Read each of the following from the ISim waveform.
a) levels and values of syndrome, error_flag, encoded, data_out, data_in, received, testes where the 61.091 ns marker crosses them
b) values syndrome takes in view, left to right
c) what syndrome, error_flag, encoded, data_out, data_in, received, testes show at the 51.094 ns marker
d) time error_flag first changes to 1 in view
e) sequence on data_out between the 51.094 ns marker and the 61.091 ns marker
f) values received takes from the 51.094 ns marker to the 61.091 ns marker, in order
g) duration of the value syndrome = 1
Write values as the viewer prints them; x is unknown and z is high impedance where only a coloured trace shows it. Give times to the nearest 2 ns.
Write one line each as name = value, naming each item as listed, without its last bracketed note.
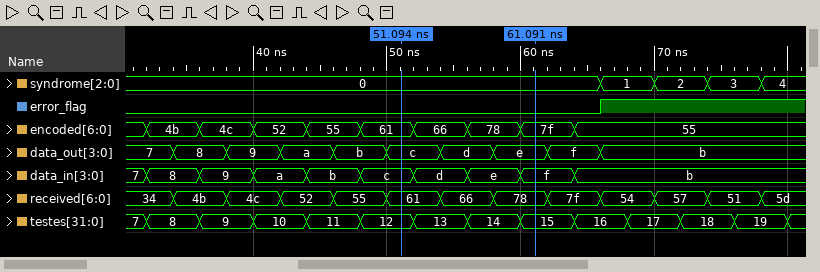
levels and values of syndrome, error_flag, encoded, data_out, data_in, received, testes where the 61.091 ns marker crosses them = syndrome=0, error_flag=0, encoded=7f, data_out=e, data_in=f, received=78, testes=15
values syndrome takes in view, left to right = 0, 1, 2, 3, 4
what syndrome, error_flag, encoded, data_out, data_in, received, testes show at the 51.094 ns marker = syndrome=0, error_flag=0, encoded=61, data_out=c, data_in=c, received=61, testes=12
time error_flag first changes to 1 in view = 66 ns
sequence on data_out between the 51.094 ns marker and the 61.091 ns marker = c, d, e
values received takes from the 51.094 ns marker to the 61.091 ns marker, in order = 61, 66, 78
duration of the value syndrome = 1 = 4 ns
